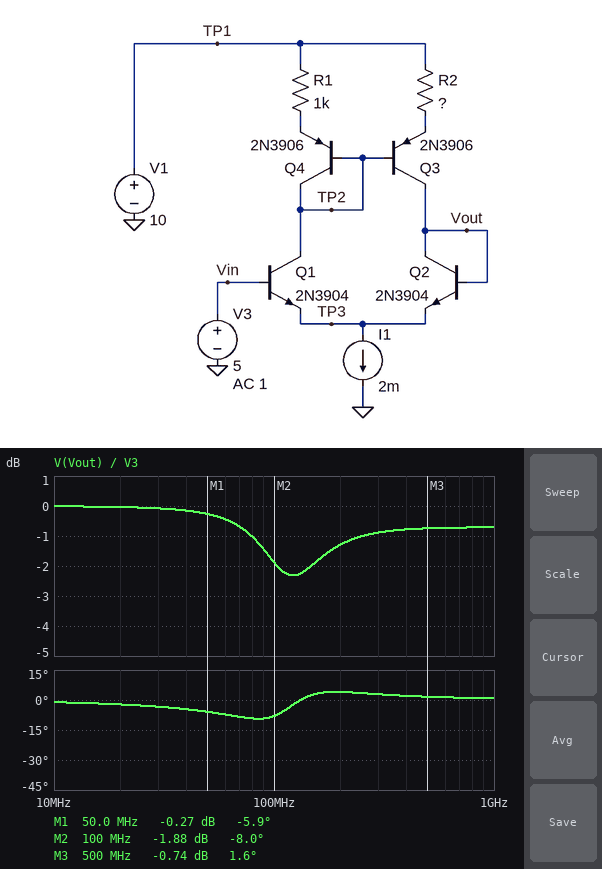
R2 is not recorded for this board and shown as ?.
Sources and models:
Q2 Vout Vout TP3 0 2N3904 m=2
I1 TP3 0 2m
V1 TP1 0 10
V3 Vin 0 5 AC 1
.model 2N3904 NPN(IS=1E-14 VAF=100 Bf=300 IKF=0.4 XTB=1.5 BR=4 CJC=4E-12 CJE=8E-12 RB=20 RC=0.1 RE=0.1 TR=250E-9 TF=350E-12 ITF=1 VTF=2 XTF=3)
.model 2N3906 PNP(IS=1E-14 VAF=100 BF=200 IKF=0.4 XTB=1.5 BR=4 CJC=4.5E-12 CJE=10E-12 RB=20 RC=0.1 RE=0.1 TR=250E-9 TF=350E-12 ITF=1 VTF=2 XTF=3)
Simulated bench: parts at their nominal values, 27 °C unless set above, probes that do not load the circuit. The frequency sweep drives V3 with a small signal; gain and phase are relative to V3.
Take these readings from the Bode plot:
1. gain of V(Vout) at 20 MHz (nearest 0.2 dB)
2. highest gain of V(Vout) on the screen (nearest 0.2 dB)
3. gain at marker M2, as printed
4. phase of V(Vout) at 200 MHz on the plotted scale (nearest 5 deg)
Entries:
0 dB
0 dB
-1.88 dB
5 deg
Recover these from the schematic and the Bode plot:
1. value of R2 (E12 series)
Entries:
390 Ω
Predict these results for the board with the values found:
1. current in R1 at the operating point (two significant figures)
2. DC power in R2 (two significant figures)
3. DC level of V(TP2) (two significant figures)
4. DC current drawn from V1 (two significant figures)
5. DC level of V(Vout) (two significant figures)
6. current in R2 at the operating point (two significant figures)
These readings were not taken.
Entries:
580 µA
790 µW
8.8 V
2.0 mA
5.0 V
1.4 mA
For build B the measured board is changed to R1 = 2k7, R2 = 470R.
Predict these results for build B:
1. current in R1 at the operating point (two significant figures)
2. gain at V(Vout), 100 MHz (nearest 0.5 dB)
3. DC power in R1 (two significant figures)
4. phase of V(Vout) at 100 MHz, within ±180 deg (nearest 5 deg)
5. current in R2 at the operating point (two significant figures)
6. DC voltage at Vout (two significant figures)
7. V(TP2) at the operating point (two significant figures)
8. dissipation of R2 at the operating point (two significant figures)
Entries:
310 µA
-2.5 dB
260 µW
5 deg
1.7 mA
5.0 V
8.5 V
1.3 mW
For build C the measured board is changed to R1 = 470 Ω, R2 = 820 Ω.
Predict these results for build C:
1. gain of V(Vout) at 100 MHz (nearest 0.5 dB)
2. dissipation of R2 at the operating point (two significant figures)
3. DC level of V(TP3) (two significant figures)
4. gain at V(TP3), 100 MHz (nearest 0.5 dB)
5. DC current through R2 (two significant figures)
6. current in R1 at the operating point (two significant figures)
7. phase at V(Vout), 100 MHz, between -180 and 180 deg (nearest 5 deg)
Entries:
-1.0 dB
450 µW
4.3 V
-0.5 dB
740 µA
1.3 mA
-5 deg
